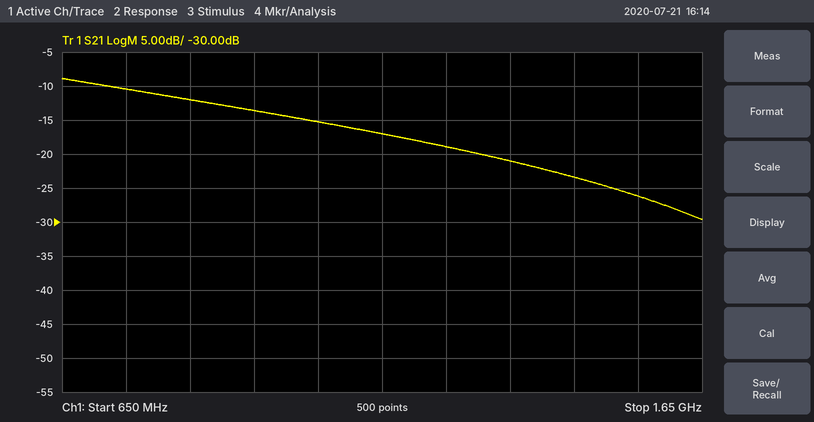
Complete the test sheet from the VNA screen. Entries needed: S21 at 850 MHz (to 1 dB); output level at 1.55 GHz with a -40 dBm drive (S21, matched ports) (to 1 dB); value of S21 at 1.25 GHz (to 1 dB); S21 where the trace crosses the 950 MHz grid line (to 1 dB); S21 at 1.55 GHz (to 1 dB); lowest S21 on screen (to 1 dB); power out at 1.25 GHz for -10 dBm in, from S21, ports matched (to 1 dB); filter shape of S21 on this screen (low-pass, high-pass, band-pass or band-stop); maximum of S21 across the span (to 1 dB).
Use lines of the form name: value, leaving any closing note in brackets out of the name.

S21 at 850 MHz: -12 dB
output level at 1.55 GHz with a -40 dBm drive (S21, matched ports): -66 dBm
value of S21 at 1.25 GHz: -19 dB
S21 where the trace crosses the 950 MHz grid line: -14 dB
S21 at 1.55 GHz: -26 dB
lowest S21 on screen: -30 dB
power out at 1.25 GHz for -10 dBm in, from S21, ports matched: -29 dBm
filter shape of S21 on this screen: low-pass
maximum of S21 across the span: -9 dB
